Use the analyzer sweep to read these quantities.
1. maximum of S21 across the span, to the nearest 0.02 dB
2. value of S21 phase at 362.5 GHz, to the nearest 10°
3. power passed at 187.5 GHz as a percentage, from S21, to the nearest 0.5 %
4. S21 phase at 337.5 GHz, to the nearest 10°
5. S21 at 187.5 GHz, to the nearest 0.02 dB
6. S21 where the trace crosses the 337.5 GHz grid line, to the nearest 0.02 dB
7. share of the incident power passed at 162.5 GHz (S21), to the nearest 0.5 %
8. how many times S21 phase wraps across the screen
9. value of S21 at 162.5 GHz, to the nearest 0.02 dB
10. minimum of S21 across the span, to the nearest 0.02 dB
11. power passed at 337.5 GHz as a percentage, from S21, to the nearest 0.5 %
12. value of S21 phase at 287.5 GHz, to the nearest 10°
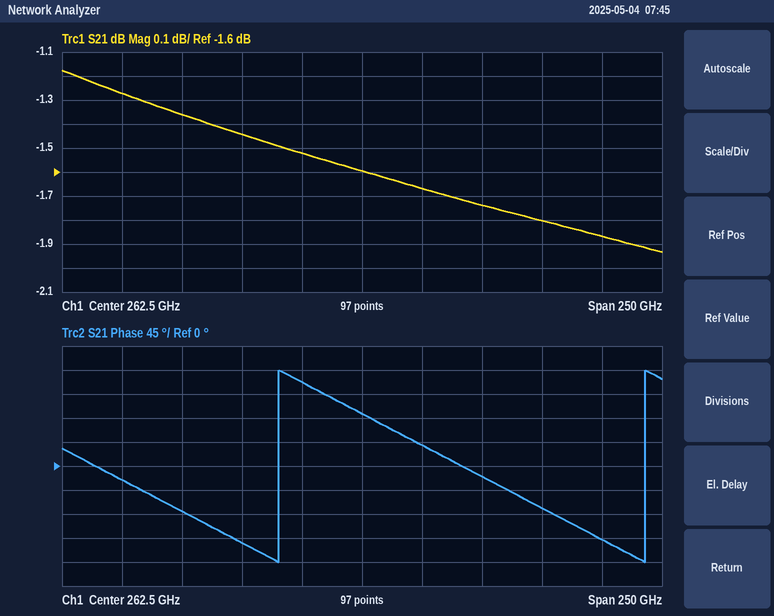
-1.18 dB
-140°
73.0 %
-80°
-1.36 dB
-1.80 dB
74.5 %
2
-1.28 dB
-1.94 dB
66.0 %
40°
